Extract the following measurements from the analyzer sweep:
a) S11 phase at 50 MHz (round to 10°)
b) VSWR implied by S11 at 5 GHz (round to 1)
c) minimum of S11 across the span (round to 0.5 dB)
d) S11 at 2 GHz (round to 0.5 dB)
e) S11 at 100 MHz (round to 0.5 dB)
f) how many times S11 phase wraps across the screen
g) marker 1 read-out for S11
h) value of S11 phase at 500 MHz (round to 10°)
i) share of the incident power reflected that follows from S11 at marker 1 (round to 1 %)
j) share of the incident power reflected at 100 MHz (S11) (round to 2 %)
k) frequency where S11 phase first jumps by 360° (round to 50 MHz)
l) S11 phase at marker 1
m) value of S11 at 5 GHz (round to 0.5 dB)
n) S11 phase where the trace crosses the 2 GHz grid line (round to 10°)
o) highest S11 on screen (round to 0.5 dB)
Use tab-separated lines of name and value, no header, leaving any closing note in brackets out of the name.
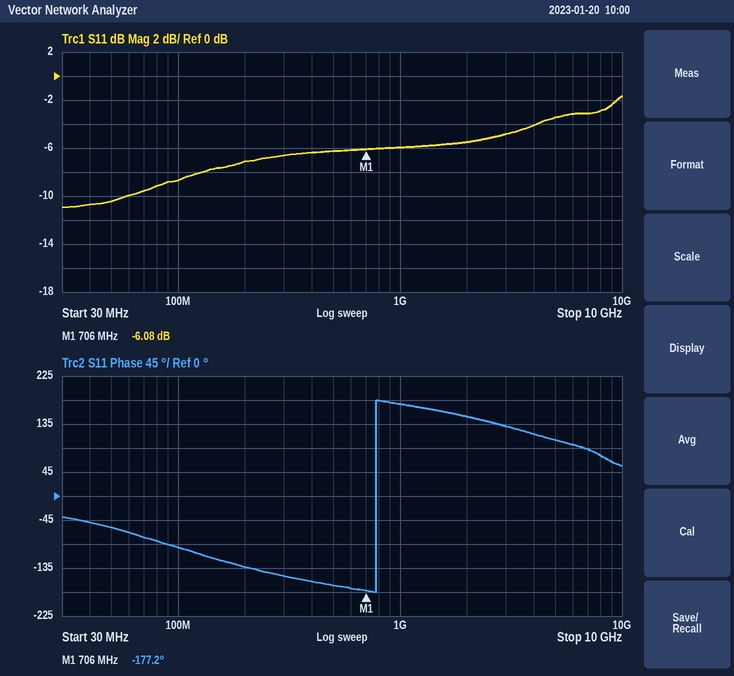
S11 phase at 50 MHz	-60°
VSWR implied by S11 at 5 GHz	5
minimum of S11 across the span	-11.0 dB
S11 at 2 GHz	-5.5 dB
S11 at 100 MHz	-8.5 dB
how many times S11 phase wraps across the screen	1
marker 1 read-out for S11	-6.08 dB
value of S11 phase at 500 MHz	-170°
share of the incident power reflected that follows from S11 at marker 1	25 %
share of the incident power reflected at 100 MHz (S11)	14 %
frequency where S11 phase first jumps by 360°	800 MHz
S11 phase at marker 1	-177.2°
value of S11 at 5 GHz	-3.5 dB
S11 phase where the trace crosses the 2 GHz grid line	150°
highest S11 on screen	-1.5 dB
